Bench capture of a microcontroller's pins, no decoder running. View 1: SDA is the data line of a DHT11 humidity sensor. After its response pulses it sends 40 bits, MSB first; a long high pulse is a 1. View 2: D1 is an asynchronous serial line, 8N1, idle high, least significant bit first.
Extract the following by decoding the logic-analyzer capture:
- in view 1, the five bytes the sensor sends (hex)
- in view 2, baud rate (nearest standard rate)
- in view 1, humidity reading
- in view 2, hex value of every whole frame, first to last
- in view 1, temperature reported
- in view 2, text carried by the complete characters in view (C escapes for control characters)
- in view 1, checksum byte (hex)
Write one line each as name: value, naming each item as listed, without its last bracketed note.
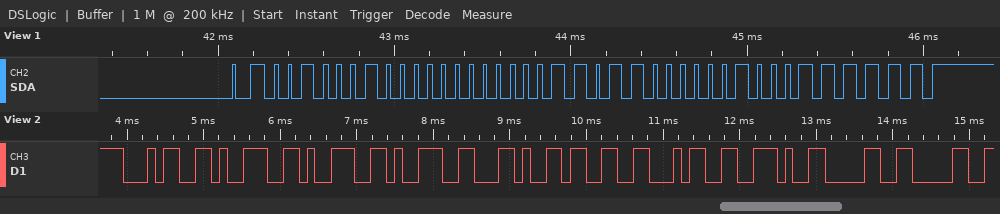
in view 1, the five bytes the sensor sends: 22 00 1B 02 3F
in view 2, baud rate: 9600 baud
in view 1, humidity reading: 34 %
in view 2, hex value of every whole frame, first to last: 34 39 39 39 2C 33 34 2E 30 30
in view 1, temperature reported: 27.2 °C
in view 2, text carried by the complete characters in view: "4999,34.00"
in view 1, checksum byte: 0x3F
